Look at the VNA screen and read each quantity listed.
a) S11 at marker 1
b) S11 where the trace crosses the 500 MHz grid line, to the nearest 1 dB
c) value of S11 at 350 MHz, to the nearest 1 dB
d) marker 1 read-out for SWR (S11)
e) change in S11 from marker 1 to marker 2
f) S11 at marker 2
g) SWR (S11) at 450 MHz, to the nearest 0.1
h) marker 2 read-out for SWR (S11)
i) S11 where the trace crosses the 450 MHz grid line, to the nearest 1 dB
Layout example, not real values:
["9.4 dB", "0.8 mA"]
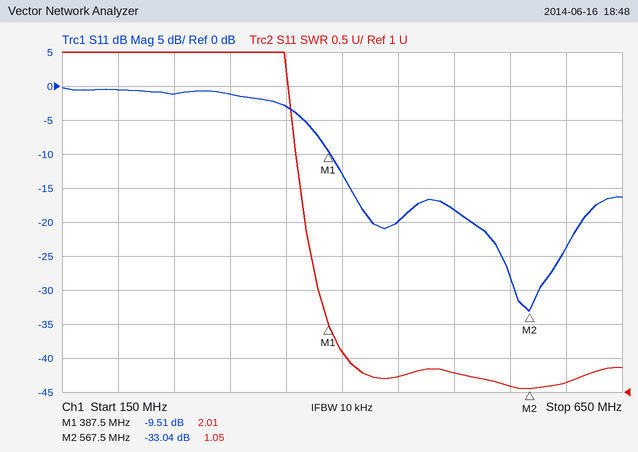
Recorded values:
["-9.51 dB", "-18 dB", "-3 dB", "2.01", "-23.53 dB", "-33.04 dB", "1.2", "1.05", "-20 dB"]
